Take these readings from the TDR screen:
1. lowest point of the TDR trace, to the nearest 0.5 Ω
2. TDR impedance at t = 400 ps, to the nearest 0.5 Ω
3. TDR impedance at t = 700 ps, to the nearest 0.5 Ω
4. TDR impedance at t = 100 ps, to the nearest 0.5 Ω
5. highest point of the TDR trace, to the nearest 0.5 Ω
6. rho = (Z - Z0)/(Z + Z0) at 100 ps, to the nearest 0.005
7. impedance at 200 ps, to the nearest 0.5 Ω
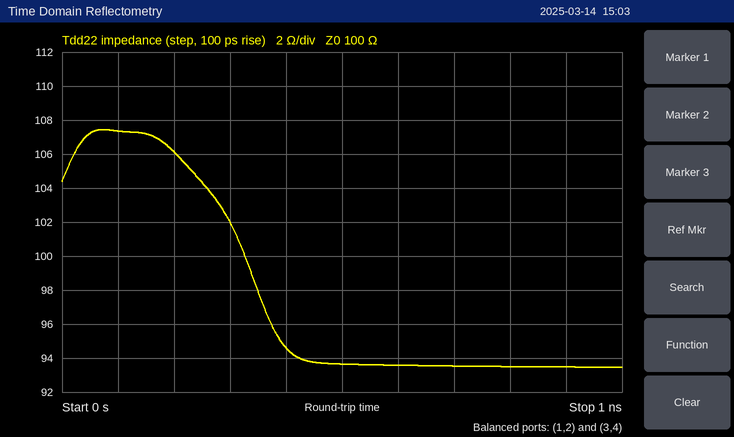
93.5 Ω
94.5 Ω
93.5 Ω
107.5 Ω
107.5 Ω
+0.035
106.0 Ω
